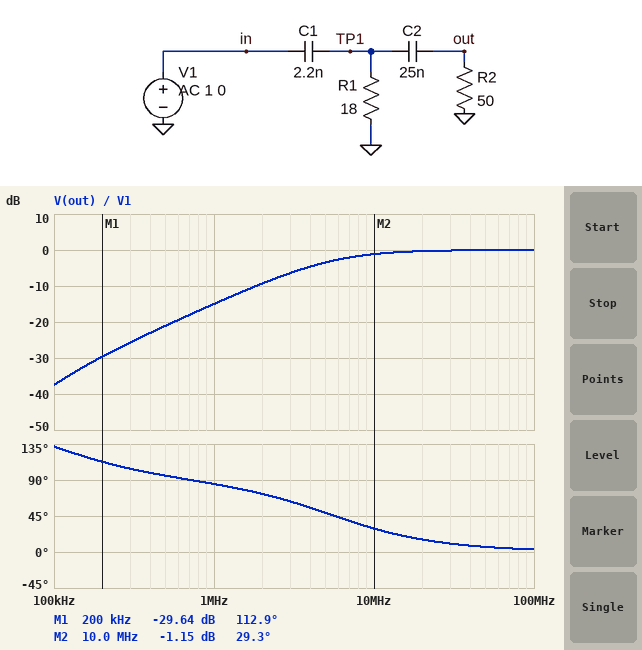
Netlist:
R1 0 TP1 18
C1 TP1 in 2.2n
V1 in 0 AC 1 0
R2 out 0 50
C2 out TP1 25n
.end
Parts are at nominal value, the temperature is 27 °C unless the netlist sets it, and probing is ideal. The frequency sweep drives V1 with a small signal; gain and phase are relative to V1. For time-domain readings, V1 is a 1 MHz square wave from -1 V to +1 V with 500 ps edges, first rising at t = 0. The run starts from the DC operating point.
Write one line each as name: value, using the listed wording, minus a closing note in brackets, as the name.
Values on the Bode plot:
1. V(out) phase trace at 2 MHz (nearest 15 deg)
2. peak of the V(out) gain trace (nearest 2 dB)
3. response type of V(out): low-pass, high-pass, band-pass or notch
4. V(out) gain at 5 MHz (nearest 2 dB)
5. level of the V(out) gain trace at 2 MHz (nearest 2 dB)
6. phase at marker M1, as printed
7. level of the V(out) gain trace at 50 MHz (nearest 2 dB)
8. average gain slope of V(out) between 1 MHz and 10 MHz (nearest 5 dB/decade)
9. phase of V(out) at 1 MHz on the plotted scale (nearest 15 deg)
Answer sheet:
V(out) phase trace at 2 MHz: 75 deg
peak of the V(out) gain trace: 0 dB
response type of V(out): low-pass, high-pass, band-pass or notch: high-pass
V(out) gain at 5 MHz: -4 dB
level of the V(out) gain trace at 2 MHz: -10 dB
phase at marker M1, as printed: 112.9 deg
level of the V(out) gain trace at 50 MHz: 0 dB
average gain slope of V(out) between 1 MHz and 10 MHz: 15 dB/decade
phase of V(out) at 1 MHz on the plotted scale: 90 deg
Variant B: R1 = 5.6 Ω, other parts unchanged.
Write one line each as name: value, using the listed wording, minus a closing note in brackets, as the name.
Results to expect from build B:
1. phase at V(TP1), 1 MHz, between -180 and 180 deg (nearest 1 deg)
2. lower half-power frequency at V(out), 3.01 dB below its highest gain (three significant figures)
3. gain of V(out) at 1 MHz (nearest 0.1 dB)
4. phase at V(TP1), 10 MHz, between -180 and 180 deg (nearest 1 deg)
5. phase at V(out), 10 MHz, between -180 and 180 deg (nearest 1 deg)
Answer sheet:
phase at V(TP1), 1 MHz, between -180 and 180 deg: 85 deg
lower half-power frequency at V(out), 3.01 dB below its highest gain: 14.4 MHz
gain of V(out) at 1 MHz: -23.2 dB
phase at V(TP1), 10 MHz, between -180 and 180 deg: 55 deg
phase at V(out), 10 MHz, between -180 and 180 deg: 56 deg
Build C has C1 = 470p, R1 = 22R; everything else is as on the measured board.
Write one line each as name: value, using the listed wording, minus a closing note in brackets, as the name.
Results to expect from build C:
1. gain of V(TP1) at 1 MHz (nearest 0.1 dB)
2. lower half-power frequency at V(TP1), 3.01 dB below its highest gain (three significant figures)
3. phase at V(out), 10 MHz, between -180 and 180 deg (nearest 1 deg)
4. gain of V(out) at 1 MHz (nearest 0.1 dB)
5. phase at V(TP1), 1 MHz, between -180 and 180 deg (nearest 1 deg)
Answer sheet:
gain of V(TP1) at 1 MHz: -26.9 dB
lower half-power frequency at V(TP1), 3.01 dB below its highest gain: 22.2 MHz
phase at V(out), 10 MHz, between -180 and 180 deg: 66 deg
gain of V(out) at 1 MHz: -27.0 dB
phase at V(TP1), 1 MHz, between -180 and 180 deg: 85 deg
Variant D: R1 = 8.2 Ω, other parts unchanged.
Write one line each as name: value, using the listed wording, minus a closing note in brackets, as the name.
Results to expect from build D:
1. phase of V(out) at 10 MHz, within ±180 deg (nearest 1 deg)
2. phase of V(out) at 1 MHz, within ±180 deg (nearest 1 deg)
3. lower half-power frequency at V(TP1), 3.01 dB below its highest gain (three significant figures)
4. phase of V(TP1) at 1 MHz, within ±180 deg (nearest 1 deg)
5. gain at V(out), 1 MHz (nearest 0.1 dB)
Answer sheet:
phase of V(out) at 10 MHz, within ±180 deg: 46 deg
phase of V(out) at 1 MHz, within ±180 deg: 91 deg
lower half-power frequency at V(TP1), 3.01 dB below its highest gain: 10.3 MHz
phase of V(TP1) at 1 MHz, within ±180 deg: 83 deg
gain at V(out), 1 MHz: -20.3 dB
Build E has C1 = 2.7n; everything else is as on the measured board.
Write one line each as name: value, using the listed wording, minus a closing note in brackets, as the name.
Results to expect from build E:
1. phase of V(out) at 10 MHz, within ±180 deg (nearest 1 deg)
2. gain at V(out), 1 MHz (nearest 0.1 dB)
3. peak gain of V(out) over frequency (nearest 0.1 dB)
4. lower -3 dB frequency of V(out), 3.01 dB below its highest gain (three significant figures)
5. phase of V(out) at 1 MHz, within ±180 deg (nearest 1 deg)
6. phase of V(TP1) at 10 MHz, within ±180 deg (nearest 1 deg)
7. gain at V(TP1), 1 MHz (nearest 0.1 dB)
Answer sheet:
phase of V(out) at 10 MHz, within ±180 deg: 25 deg
gain at V(out), 1 MHz: -13.3 dB
peak gain of V(out) over frequency: 0 dB
lower -3 dB frequency of V(out), 3.01 dB below its highest gain: 4.49 MHz
phase of V(out) at 1 MHz, within ±180 deg: 83 deg
phase of V(TP1) at 10 MHz, within ±180 deg: 24 deg
gain at V(TP1), 1 MHz: -13.2 dB
